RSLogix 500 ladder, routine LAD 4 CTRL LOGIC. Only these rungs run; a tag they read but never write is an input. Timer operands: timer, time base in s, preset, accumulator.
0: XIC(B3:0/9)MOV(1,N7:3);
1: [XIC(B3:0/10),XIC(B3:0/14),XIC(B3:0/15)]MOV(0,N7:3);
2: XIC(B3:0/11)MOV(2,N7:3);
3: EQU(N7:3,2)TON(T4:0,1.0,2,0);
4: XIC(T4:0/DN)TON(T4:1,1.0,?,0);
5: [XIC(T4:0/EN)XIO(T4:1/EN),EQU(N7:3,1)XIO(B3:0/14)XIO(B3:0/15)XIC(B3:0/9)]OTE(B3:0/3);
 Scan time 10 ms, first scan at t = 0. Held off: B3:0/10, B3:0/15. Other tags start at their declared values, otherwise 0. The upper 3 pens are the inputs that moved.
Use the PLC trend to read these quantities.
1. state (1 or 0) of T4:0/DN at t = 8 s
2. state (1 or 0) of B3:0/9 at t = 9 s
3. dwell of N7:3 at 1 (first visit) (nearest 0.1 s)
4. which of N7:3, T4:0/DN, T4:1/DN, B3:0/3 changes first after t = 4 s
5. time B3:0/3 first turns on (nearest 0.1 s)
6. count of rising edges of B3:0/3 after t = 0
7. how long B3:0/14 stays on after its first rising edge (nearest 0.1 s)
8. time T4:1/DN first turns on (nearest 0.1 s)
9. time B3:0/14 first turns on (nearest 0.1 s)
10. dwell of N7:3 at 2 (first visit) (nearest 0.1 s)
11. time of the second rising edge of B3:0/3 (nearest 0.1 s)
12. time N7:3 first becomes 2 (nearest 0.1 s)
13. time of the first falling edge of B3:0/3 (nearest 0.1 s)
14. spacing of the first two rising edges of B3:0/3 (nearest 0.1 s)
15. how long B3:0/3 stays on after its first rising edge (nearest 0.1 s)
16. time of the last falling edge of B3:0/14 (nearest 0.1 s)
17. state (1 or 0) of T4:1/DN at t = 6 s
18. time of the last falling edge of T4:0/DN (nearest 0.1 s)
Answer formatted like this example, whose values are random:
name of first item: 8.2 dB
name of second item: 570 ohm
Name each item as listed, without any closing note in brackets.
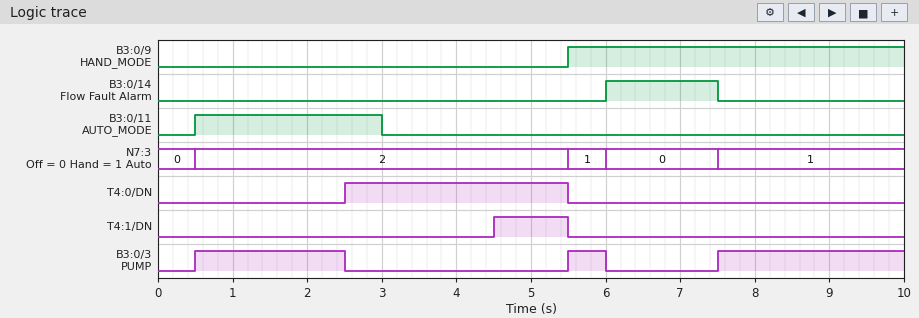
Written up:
state (1 or 0) of T4:0/DN at t = 8 s: 0
state (1 or 0) of B3:0/9 at t = 9 s: 1
dwell of N7:3 at 1 (first visit): 0.5 s
which of N7:3, T4:0/DN, T4:1/DN, B3:0/3 changes first after t = 4 s: T4:1/DN
time B3:0/3 first turns on: 0.5 s
count of rising edges of B3:0/3 after t = 0: 3
how long B3:0/14 stays on after its first rising edge: 1.5 s
time T4:1/DN first turns on: 4.5 s
time B3:0/14 first turns on: 6.0 s
dwell of N7:3 at 2 (first visit): 5.0 s
time of the second rising edge of B3:0/3: 5.5 s
time N7:3 first becomes 2: 0.5 s
time of the first falling edge of B3:0/3: 2.5 s
spacing of the first two rising edges of B3:0/3: 5.0 s
how long B3:0/3 stays on after its first rising edge: 2.0 s
time of the last falling edge of B3:0/14: 7.5 s
state (1 or 0) of T4:1/DN at t = 6 s: 0
time of the last falling edge of T4:0/DN: 5.5 s
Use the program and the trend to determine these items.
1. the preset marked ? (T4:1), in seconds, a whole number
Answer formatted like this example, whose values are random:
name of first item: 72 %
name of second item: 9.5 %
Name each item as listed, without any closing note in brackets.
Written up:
the preset marked ? (T4:1), in seconds, a whole number: 2 s
